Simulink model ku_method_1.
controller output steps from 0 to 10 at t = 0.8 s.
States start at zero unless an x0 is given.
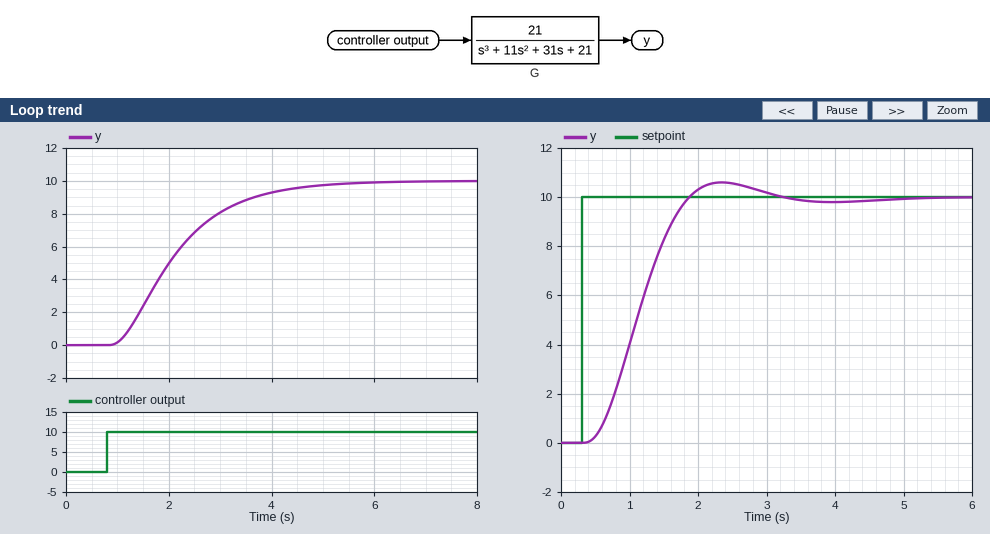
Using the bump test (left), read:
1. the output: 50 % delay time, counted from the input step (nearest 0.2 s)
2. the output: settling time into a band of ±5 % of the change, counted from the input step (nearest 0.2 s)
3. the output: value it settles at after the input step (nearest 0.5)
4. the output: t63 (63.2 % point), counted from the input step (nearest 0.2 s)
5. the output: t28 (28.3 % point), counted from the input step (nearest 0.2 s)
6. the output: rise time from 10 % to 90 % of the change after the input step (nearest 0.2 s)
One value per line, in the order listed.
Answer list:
1.2 s
3.6 s
10.0
1.6 s
0.8 s
2.4 s
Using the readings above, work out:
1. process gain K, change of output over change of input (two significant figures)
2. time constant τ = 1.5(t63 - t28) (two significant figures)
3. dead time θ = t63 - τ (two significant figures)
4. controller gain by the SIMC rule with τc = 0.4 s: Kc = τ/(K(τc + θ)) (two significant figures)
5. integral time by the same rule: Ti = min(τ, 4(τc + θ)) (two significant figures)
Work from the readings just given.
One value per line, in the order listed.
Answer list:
1.0
1.2 s
0.40 s
1.5
1.2 s
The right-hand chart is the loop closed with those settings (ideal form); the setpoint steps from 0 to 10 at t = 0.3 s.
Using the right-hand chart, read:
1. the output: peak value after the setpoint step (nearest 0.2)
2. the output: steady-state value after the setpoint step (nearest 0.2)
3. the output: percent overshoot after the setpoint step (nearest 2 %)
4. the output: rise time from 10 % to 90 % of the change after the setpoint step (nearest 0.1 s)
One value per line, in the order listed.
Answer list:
10.6
10.0
6 %
1.0 s
